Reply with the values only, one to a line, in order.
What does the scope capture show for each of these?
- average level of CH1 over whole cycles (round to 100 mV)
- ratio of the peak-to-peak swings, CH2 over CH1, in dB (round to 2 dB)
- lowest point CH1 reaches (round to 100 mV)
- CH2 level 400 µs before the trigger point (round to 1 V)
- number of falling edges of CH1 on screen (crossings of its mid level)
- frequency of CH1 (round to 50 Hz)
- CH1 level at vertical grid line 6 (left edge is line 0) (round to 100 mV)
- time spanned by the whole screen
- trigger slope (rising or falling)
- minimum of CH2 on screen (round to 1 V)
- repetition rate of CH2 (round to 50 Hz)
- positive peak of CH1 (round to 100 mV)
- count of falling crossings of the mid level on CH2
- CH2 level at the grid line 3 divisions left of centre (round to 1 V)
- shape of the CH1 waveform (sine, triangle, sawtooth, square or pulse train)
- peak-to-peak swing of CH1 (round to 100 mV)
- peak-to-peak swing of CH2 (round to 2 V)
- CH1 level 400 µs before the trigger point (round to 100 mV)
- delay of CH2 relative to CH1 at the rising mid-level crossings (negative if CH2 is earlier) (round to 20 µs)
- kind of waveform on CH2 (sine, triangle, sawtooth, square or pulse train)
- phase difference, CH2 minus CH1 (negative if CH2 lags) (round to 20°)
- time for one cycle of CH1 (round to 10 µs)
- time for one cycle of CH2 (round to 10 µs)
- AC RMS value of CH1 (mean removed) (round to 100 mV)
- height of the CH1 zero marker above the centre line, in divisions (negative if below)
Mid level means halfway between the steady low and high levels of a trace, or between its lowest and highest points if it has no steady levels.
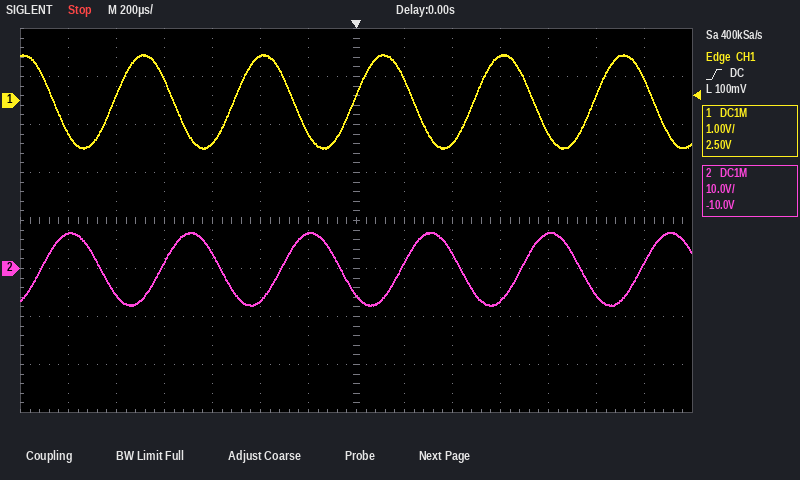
0.0 V
18 dB
-1.0 V
-7 V
6
2.00 kHz
-700 mV
2.8 ms
rising
-8 V
2.00 kHz
1.0 V
5
3 V
sine
2.0 V
16 V
900 mV
+200 µs
sine
-140°
500 µs
500 µs
700 mV
+2.5 div
